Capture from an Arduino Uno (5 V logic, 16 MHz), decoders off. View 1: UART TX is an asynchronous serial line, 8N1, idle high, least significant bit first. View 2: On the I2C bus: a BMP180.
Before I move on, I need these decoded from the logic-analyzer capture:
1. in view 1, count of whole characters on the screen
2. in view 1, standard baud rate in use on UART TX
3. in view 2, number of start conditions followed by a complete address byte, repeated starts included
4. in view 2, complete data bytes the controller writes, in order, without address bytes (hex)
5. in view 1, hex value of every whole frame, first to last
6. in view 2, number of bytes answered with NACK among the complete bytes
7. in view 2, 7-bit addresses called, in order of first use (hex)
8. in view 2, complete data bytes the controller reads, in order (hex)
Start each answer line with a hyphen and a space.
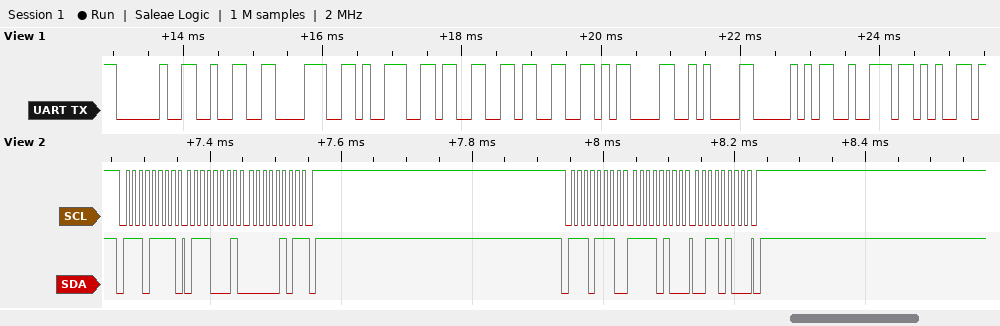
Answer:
- 11
- 9600 baud
- 2
- F4 34
- 20 32 38 39 33 33 0D 0A 50 72 65
- 1
- 0x77
- 71 05
